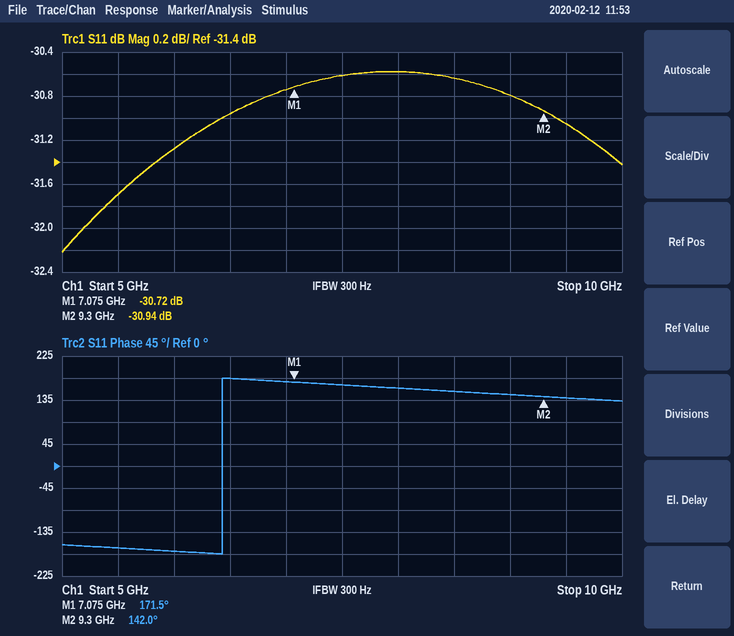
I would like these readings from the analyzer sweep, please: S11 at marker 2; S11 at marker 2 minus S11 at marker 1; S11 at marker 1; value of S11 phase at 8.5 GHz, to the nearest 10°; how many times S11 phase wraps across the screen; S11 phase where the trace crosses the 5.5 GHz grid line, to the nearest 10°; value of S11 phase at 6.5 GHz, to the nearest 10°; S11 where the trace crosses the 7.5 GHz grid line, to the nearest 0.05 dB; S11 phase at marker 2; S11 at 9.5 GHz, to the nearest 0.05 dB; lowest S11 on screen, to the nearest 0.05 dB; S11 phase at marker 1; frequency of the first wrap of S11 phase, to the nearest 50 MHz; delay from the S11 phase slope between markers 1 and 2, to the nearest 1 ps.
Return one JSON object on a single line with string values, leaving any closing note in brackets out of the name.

{"S11 at marker 2": "-30.94 dB", "S11 at marker 2 minus S11 at marker 1": "-0.22 dB", "S11 at marker 1": "-30.72 dB", "value of S11 phase at 8.5 GHz, to the nearest 10°": "150°", "how many times S11 phase wraps across the screen": "1", "S11 phase where the trace crosses the 5.5 GHz grid line, to the nearest 10°": "-170°", "value of S11 phase at 6.5 GHz, to the nearest 10°": "180°", "S11 where the trace crosses the 7.5 GHz grid line, to the nearest 0.05 dB": "-30.60 dB", "S11 phase at marker 2": "142.0°", "S11 at 9.5 GHz, to the nearest 0.05 dB": "-31.05 dB", "lowest S11 on screen, to the nearest 0.05 dB": "-32.20 dB", "S11 phase at marker 1": "171.5°", "frequency of the first wrap of S11 phase, to the nearest 50 MHz": "6.45 GHz", "delay from the S11 phase slope between markers 1 and 2, to the nearest 1 ps": "37 ps"}
